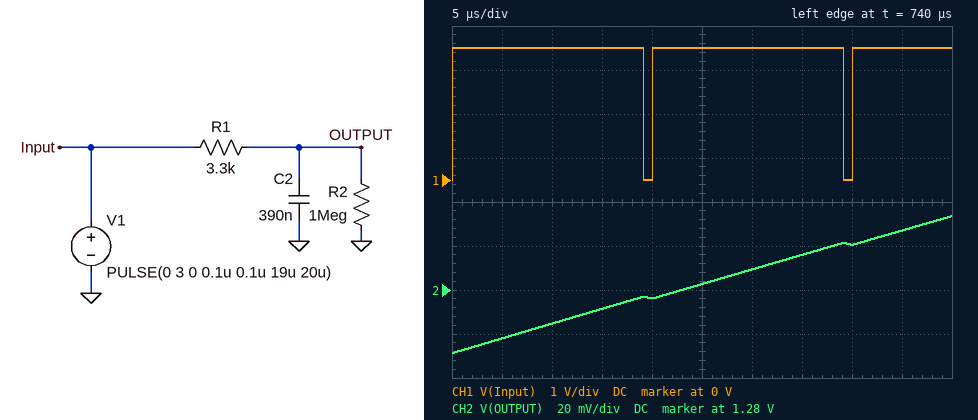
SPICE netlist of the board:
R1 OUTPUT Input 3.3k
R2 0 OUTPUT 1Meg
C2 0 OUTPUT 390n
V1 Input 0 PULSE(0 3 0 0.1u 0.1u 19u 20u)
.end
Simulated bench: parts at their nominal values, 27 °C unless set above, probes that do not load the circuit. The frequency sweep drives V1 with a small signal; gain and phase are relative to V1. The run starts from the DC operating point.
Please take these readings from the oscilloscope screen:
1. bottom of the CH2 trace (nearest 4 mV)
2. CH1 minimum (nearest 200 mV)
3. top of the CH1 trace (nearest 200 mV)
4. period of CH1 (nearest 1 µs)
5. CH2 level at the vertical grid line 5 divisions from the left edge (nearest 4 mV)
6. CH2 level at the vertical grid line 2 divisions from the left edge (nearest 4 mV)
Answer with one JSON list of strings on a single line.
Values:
["1.252 V", "0 V", "3.0 V", "20 µs", "1.284 V", "1.264 V"]
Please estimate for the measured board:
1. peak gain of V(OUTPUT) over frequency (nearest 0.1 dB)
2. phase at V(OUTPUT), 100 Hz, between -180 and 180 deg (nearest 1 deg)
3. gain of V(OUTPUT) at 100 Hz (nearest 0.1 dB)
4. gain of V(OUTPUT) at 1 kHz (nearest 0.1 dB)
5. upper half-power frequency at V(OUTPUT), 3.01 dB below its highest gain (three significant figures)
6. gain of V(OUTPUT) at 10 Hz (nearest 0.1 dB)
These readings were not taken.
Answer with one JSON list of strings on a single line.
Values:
["0 dB", "-39 deg", "-2.2 dB", "-18.2 dB", "124 Hz", "-0.1 dB"]
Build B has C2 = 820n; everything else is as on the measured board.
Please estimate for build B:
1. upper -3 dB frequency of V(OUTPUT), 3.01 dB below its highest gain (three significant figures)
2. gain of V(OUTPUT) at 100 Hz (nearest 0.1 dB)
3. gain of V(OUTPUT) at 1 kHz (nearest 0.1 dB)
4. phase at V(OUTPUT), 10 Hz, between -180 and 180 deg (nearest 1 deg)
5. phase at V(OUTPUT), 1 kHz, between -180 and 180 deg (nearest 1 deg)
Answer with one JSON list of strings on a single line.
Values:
["59.0 Hz", "-5.9 dB", "-24.6 dB", "-10 deg", "-87 deg"]
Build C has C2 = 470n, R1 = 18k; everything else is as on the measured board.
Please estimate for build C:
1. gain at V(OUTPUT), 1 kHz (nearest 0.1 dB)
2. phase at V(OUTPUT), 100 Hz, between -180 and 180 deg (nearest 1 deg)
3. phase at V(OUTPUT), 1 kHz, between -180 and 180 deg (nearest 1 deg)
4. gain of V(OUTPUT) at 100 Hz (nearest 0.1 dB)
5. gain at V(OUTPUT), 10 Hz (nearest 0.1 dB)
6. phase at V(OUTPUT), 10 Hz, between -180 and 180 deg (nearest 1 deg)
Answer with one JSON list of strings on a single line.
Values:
["-34.5 dB", "-79 deg", "-89 deg", "-14.7 dB", "-1.2 dB", "-28 deg"]
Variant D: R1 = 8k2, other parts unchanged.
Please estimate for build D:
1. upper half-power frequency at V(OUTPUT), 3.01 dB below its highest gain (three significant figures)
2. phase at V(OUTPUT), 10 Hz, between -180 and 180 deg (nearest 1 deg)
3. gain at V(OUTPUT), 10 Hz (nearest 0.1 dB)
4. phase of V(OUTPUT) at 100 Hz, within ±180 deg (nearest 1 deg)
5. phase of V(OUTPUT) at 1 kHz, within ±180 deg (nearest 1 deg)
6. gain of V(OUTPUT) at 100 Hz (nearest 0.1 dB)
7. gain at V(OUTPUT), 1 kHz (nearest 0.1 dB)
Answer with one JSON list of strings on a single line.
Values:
["50.2 Hz", "-11 deg", "-0.2 dB", "-63 deg", "-87 deg", "-7.0 dB", "-26.1 dB"]
